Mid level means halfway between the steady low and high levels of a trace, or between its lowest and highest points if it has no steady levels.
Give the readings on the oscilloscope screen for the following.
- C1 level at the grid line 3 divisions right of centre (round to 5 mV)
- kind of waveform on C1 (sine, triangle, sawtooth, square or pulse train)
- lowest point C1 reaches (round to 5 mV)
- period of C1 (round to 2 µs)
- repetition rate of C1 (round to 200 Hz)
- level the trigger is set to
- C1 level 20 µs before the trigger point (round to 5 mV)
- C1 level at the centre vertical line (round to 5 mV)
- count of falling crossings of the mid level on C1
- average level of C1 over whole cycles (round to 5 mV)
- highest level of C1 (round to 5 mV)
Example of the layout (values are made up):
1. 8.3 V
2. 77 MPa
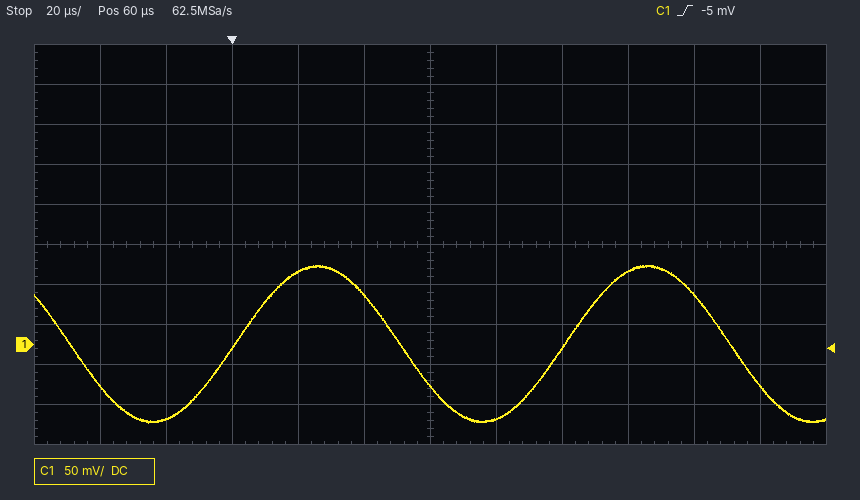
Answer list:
1. 90 mV
2. sine
3. -100 mV
4. 100 µs
5. 10.0 kHz
6. -5 mV
7. -95 mV
8. -50 mV
9. 3
10. 0 mV
11. 100 mV
